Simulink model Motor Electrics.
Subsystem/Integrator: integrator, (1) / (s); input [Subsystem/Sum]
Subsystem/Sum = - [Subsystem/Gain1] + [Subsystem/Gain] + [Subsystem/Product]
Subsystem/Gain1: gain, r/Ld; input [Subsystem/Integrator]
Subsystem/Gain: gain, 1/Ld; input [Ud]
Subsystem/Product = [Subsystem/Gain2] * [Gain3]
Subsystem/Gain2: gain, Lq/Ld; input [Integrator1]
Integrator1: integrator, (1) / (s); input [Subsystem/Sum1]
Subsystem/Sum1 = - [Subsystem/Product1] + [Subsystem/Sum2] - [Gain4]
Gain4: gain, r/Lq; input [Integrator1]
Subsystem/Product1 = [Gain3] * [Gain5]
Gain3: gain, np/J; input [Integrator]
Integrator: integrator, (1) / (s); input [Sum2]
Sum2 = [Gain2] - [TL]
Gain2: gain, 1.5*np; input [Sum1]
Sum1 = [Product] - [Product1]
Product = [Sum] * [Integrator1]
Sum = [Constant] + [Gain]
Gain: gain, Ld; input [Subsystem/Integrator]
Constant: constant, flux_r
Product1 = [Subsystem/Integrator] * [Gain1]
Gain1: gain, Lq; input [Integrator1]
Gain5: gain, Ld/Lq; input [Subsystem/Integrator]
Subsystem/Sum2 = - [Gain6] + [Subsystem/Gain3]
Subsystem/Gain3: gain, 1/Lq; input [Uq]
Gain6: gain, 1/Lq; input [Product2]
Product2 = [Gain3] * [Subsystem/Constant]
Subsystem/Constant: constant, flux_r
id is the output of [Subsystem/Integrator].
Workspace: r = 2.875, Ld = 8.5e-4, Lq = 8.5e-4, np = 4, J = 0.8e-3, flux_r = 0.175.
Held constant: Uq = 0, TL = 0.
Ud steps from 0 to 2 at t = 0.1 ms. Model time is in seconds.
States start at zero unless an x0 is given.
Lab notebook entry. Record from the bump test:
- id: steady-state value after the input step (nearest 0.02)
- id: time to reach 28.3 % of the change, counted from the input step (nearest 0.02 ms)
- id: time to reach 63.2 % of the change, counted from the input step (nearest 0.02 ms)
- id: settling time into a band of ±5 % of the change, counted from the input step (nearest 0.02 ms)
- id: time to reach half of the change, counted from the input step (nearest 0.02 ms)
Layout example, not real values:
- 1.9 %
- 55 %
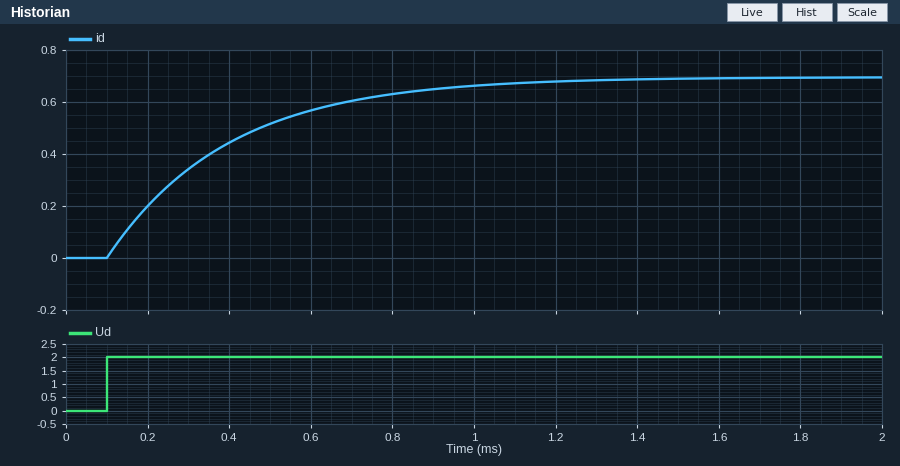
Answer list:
- 0.70
- 0.10 ms
- 0.30 ms
- 0.88 ms
- 0.20 ms
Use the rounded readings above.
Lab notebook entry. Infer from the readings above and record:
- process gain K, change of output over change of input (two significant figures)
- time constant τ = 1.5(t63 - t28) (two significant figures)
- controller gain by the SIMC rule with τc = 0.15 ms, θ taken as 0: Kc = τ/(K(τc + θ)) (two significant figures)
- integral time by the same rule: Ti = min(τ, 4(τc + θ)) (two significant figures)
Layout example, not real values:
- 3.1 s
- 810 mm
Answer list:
- 0.35
- 0.30 ms
- 5.7
- 0.30 ms
